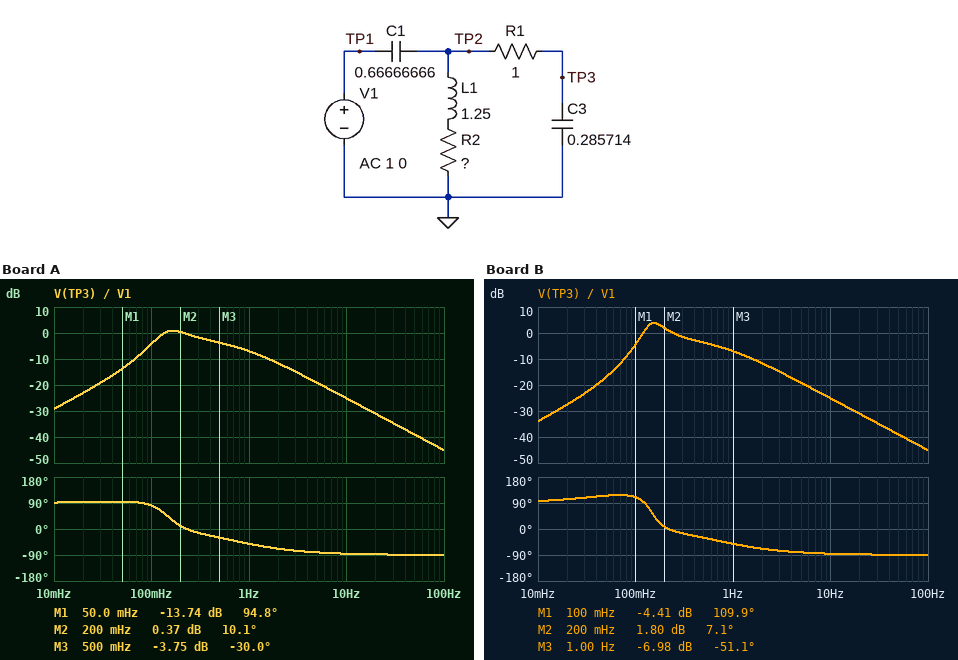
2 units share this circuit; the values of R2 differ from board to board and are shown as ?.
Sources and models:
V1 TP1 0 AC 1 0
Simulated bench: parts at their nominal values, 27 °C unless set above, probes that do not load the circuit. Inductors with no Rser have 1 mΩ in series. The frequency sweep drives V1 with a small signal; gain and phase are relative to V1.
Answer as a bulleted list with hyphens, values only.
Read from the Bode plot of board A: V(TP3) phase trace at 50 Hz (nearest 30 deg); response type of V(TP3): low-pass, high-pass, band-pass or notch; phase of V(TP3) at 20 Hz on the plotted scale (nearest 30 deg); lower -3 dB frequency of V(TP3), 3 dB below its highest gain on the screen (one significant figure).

- -90 deg
- band-pass
- -90 deg
- 100 mHz
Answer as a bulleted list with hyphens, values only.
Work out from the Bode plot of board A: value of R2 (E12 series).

- 0.82 Ω
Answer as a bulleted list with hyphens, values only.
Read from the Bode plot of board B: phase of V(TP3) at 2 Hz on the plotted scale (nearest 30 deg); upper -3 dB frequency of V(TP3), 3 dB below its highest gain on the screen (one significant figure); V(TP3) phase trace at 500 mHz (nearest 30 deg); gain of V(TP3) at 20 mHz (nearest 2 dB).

- -60 deg
- 200 mHz
- -30 deg
- -28 dB
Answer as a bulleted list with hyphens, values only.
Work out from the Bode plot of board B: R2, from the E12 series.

- 0.47 Ω
